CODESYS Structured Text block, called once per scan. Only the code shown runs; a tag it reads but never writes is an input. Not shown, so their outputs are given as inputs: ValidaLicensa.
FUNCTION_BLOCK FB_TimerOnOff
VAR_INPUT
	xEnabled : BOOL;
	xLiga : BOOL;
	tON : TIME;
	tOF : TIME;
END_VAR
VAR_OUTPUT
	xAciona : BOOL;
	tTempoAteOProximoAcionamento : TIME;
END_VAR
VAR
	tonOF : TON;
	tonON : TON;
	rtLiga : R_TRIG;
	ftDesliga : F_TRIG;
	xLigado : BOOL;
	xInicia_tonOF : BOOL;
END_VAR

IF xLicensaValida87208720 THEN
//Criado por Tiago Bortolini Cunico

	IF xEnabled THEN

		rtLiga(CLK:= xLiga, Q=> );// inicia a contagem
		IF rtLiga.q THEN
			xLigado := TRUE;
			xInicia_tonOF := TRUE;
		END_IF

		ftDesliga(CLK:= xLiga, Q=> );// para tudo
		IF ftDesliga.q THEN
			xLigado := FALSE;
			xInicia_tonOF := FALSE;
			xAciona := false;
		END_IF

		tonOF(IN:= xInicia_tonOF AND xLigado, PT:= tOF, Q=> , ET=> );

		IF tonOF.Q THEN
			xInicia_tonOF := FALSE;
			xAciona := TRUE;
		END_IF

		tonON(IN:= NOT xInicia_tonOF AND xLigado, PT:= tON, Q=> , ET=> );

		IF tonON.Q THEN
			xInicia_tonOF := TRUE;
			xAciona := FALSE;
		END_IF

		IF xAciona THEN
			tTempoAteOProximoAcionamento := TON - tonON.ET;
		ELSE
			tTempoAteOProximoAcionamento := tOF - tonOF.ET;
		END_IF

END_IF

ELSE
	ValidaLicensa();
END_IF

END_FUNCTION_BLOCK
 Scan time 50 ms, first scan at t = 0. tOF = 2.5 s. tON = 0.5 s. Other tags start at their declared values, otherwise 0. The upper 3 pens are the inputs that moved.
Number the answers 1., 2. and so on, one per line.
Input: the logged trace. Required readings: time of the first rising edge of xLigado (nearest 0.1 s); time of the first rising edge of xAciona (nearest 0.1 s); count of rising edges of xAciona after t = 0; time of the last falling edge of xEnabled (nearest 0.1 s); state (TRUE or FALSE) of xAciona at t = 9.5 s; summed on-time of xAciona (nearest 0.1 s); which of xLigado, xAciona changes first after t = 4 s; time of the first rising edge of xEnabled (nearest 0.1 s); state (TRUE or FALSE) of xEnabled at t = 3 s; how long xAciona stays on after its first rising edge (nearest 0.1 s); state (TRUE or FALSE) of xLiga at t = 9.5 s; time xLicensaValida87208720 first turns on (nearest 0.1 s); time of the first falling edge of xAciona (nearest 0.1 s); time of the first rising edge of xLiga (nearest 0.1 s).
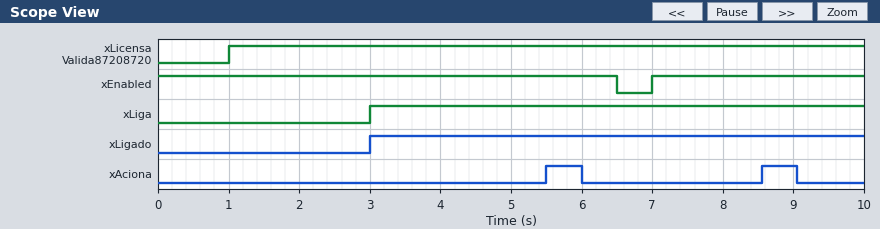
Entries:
1. 3.0 s
2. 5.5 s
3. 2
4. 6.5 s
5. FALSE
6. 1.0 s
7. xAciona
8. 7.0 s
9. TRUE
10. 0.5 s
11. TRUE
12. 1.0 s
13. 6.0 s
14. 3.0 s
